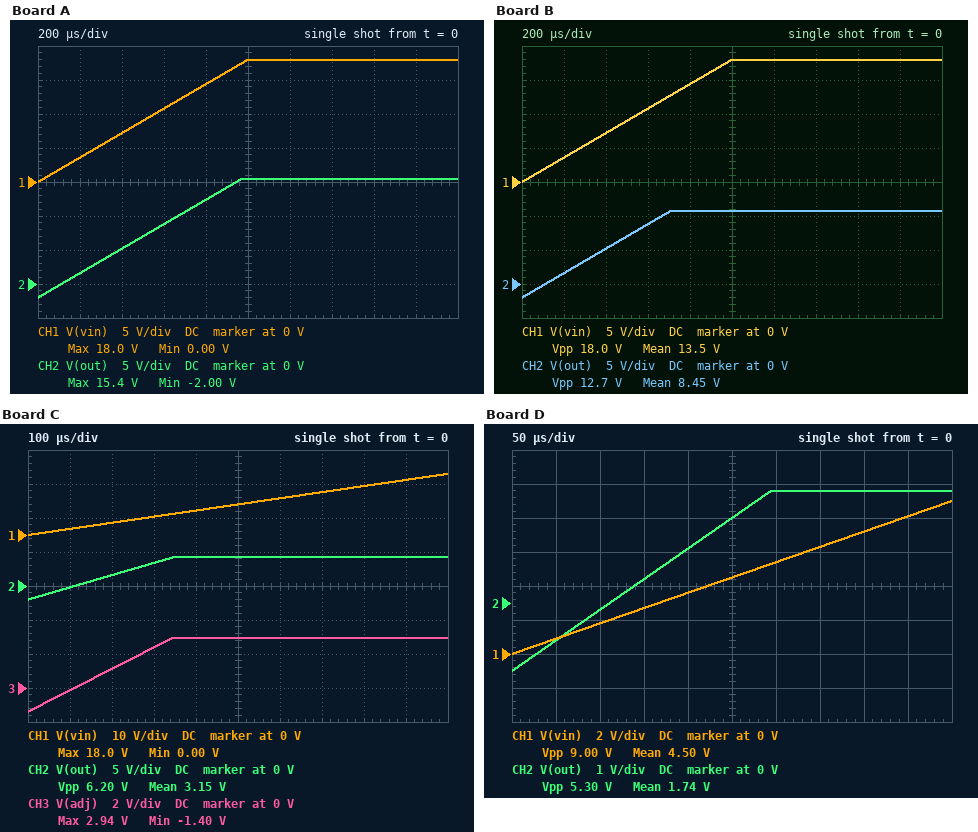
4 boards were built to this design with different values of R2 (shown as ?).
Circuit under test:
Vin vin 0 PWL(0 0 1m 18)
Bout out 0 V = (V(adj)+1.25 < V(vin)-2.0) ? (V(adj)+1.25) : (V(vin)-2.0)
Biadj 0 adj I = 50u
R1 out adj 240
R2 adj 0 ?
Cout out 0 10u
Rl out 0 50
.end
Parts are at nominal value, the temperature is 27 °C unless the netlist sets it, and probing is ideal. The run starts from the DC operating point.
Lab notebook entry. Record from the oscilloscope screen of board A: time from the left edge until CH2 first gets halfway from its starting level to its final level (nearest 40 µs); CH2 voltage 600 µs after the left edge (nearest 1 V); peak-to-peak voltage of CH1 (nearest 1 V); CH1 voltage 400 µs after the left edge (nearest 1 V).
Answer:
480 µs
9 V
18 V
7 V
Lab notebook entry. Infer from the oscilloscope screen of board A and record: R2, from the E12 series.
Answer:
2.7 kΩ
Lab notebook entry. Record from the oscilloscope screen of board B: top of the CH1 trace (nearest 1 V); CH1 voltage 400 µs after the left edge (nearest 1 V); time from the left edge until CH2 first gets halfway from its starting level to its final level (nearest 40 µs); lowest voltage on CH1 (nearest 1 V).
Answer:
18 V
7 V
360 µs
0 V
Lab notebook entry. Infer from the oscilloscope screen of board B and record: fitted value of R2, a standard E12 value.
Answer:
1.8 kΩ
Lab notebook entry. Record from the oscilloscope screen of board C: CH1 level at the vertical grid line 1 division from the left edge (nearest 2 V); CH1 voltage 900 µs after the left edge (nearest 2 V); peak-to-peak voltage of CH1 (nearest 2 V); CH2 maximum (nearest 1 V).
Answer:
2 V
16 V
18 V
4 V
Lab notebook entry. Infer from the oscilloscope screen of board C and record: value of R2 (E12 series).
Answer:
560 Ω
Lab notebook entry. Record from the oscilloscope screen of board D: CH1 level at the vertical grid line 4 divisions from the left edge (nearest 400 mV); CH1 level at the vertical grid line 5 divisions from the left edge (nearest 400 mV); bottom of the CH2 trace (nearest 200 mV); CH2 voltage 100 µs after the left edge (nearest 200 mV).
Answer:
3.6 V
4.4 V
-2.0 V
-200 mV
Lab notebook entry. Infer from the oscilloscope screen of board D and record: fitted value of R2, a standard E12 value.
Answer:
390 Ω
